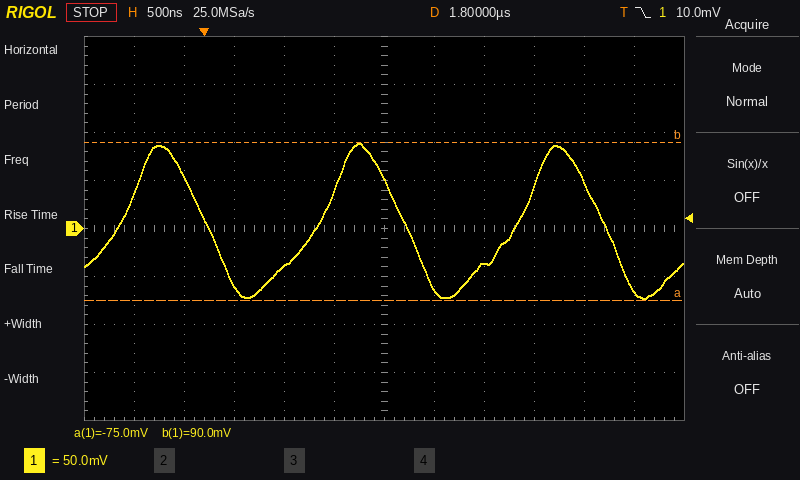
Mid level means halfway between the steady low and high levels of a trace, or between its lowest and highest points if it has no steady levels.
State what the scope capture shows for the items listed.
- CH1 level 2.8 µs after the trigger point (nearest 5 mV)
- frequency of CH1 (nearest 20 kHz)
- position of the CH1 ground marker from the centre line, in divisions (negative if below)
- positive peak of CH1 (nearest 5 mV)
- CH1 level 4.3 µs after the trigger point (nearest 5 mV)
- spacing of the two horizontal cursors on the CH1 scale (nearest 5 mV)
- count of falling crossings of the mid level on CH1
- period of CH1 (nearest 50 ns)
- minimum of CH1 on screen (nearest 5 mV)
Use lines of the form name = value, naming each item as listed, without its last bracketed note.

CH1 level 2.8 µs after the trigger point = -35 mV
frequency of CH1 = 500 kHz
position of the CH1 ground marker from the centre line, in divisions = 0.0 div
positive peak of CH1 = 90 mV
CH1 level 4.3 µs after the trigger point = -65 mV
spacing of the two horizontal cursors on the CH1 scale = 165 mV
count of falling crossings of the mid level on CH1 = 3
period of CH1 = 2.00 µs
minimum of CH1 on screen = -75 mV
